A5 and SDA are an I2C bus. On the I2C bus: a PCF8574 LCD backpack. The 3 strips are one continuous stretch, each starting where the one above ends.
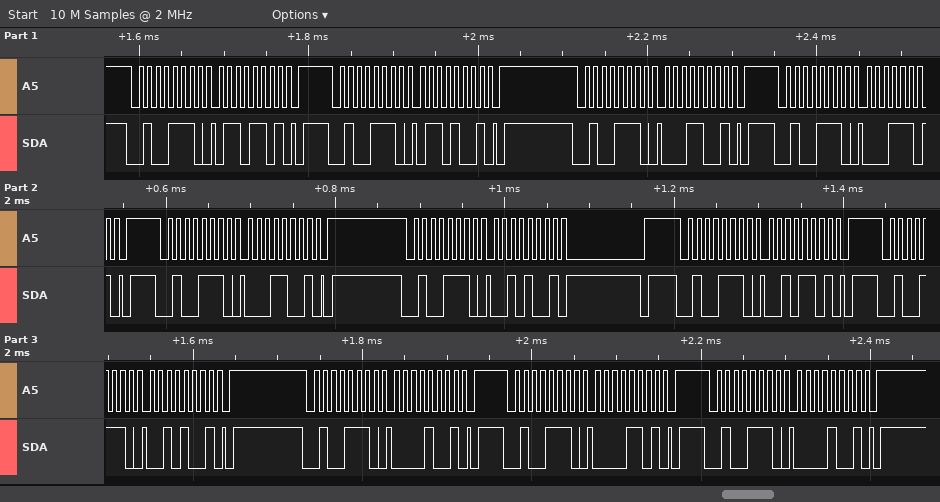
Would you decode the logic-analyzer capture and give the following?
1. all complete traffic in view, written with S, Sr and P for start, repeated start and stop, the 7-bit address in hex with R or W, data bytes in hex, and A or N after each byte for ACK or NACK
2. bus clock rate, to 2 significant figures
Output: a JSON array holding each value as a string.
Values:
["S 27W A 6D A P S 27W A 69 A P S 27W A 19 A P S 27W A 1D A P S 27W A 19 A P S 27W A 29 A P S 27W A 2D A P S 27W A 29 A P S 27W A 09 A P S 27W A 0D A P S 27W A 09 A P", "100 kHz"]
